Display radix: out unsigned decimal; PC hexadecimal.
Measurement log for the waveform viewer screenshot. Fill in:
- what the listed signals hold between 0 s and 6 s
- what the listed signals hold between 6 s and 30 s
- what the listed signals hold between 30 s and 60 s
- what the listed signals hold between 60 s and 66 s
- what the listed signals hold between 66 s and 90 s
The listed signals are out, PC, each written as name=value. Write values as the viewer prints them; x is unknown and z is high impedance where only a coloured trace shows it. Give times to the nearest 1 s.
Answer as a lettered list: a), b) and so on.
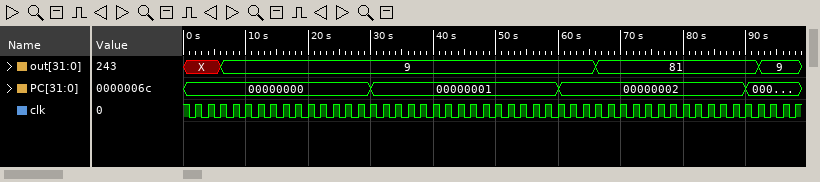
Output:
a) out=X, PC=00000000
b) out=9, PC=00000000
c) out=9, PC=00000001
d) out=9, PC=00000002
e) out=81, PC=00000002
